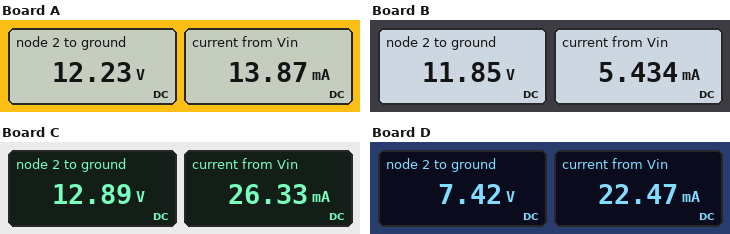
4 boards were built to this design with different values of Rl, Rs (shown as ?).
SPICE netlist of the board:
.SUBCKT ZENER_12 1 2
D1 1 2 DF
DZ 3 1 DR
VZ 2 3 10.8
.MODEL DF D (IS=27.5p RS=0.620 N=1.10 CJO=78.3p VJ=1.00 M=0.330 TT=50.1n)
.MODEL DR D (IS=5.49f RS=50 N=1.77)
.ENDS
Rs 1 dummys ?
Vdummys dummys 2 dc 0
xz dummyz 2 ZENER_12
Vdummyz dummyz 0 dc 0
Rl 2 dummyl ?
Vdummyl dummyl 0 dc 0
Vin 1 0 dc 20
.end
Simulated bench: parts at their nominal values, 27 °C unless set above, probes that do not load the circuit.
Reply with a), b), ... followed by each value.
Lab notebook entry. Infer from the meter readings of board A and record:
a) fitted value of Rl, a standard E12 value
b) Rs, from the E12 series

a) 1.2 kΩ
b) 560 Ω
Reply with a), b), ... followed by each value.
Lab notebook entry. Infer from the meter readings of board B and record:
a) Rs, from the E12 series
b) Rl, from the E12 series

a) 1.5 kΩ
b) 2.2 kΩ
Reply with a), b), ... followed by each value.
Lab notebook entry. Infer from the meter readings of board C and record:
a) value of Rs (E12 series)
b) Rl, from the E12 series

a) 270 Ω
b) 1.2 kΩ
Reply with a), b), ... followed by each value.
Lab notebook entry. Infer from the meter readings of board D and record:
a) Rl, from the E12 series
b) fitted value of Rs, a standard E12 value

a) 330 Ω
b) 560 Ω
